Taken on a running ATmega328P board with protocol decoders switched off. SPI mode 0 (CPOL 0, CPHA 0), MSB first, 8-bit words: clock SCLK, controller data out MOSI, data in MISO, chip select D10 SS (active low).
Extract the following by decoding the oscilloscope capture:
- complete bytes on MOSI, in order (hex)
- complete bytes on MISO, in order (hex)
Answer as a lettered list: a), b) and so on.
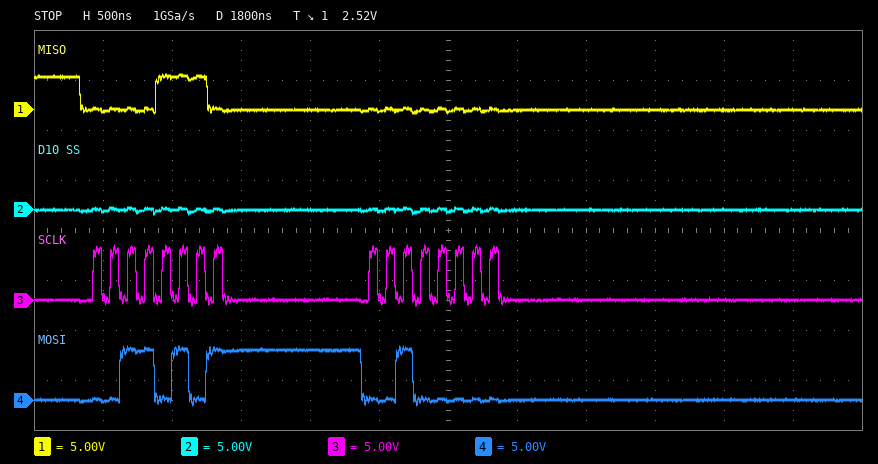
a) 0x35 0x20
b) 0x0E 0x00
